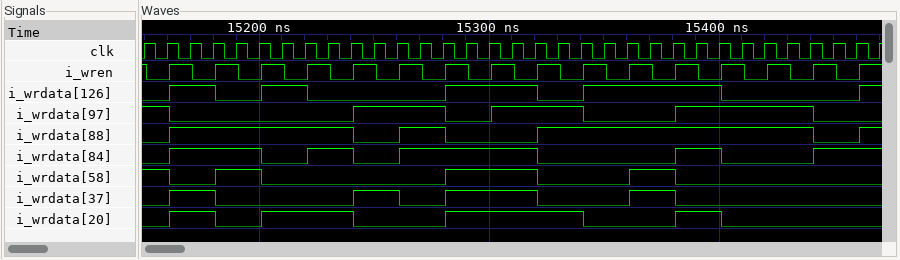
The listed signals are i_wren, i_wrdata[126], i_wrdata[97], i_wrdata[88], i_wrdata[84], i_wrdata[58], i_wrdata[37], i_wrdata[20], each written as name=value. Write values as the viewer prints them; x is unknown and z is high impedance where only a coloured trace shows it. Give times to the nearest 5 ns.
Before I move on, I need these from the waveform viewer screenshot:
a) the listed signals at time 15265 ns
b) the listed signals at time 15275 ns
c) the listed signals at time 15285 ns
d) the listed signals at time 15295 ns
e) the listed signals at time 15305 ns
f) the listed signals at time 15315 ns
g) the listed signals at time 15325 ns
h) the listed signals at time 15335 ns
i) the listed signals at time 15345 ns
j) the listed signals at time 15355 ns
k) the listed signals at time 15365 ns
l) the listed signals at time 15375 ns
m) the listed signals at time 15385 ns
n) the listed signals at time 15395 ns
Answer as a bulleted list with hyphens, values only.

- i_wren=1, i_wrdata[126]=0, i_wrdata[97]=1, i_wrdata[88]=1, i_wrdata[84]=1, i_wrdata[58]=0, i_wrdata[37]=0, i_wrdata[20]=0
- i_wren=0, i_wrdata[126]=0, i_wrdata[97]=1, i_wrdata[88]=1, i_wrdata[84]=1, i_wrdata[58]=0, i_wrdata[37]=0, i_wrdata[20]=0
- i_wren=1, i_wrdata[126]=1, i_wrdata[97]=0, i_wrdata[88]=0, i_wrdata[84]=1, i_wrdata[58]=1, i_wrdata[37]=1, i_wrdata[20]=1
- i_wren=0, i_wrdata[126]=1, i_wrdata[97]=0, i_wrdata[88]=0, i_wrdata[84]=1, i_wrdata[58]=1, i_wrdata[37]=1, i_wrdata[20]=1
- i_wren=1, i_wrdata[126]=1, i_wrdata[97]=1, i_wrdata[88]=0, i_wrdata[84]=1, i_wrdata[58]=1, i_wrdata[37]=1, i_wrdata[20]=1
- i_wren=0, i_wrdata[126]=1, i_wrdata[97]=1, i_wrdata[88]=0, i_wrdata[84]=1, i_wrdata[58]=1, i_wrdata[37]=1, i_wrdata[20]=1
- i_wren=1, i_wrdata[126]=0, i_wrdata[97]=1, i_wrdata[88]=1, i_wrdata[84]=0, i_wrdata[58]=0, i_wrdata[37]=0, i_wrdata[20]=1
- i_wren=0, i_wrdata[126]=0, i_wrdata[97]=1, i_wrdata[88]=1, i_wrdata[84]=0, i_wrdata[58]=0, i_wrdata[37]=0, i_wrdata[20]=1
- i_wren=1, i_wrdata[126]=1, i_wrdata[97]=0, i_wrdata[88]=1, i_wrdata[84]=0, i_wrdata[58]=0, i_wrdata[37]=0, i_wrdata[20]=0
- i_wren=0, i_wrdata[126]=1, i_wrdata[97]=0, i_wrdata[88]=1, i_wrdata[84]=0, i_wrdata[58]=0, i_wrdata[37]=0, i_wrdata[20]=0
- i_wren=1, i_wrdata[126]=1, i_wrdata[97]=0, i_wrdata[88]=1, i_wrdata[84]=0, i_wrdata[58]=1, i_wrdata[37]=1, i_wrdata[20]=0
- i_wren=0, i_wrdata[126]=1, i_wrdata[97]=0, i_wrdata[88]=1, i_wrdata[84]=0, i_wrdata[58]=1, i_wrdata[37]=1, i_wrdata[20]=0
- i_wren=1, i_wrdata[126]=1, i_wrdata[97]=1, i_wrdata[88]=1, i_wrdata[84]=1, i_wrdata[58]=0, i_wrdata[37]=0, i_wrdata[20]=1
- i_wren=0, i_wrdata[126]=1, i_wrdata[97]=1, i_wrdata[88]=1, i_wrdata[84]=1, i_wrdata[58]=0, i_wrdata[37]=0, i_wrdata[20]=1
